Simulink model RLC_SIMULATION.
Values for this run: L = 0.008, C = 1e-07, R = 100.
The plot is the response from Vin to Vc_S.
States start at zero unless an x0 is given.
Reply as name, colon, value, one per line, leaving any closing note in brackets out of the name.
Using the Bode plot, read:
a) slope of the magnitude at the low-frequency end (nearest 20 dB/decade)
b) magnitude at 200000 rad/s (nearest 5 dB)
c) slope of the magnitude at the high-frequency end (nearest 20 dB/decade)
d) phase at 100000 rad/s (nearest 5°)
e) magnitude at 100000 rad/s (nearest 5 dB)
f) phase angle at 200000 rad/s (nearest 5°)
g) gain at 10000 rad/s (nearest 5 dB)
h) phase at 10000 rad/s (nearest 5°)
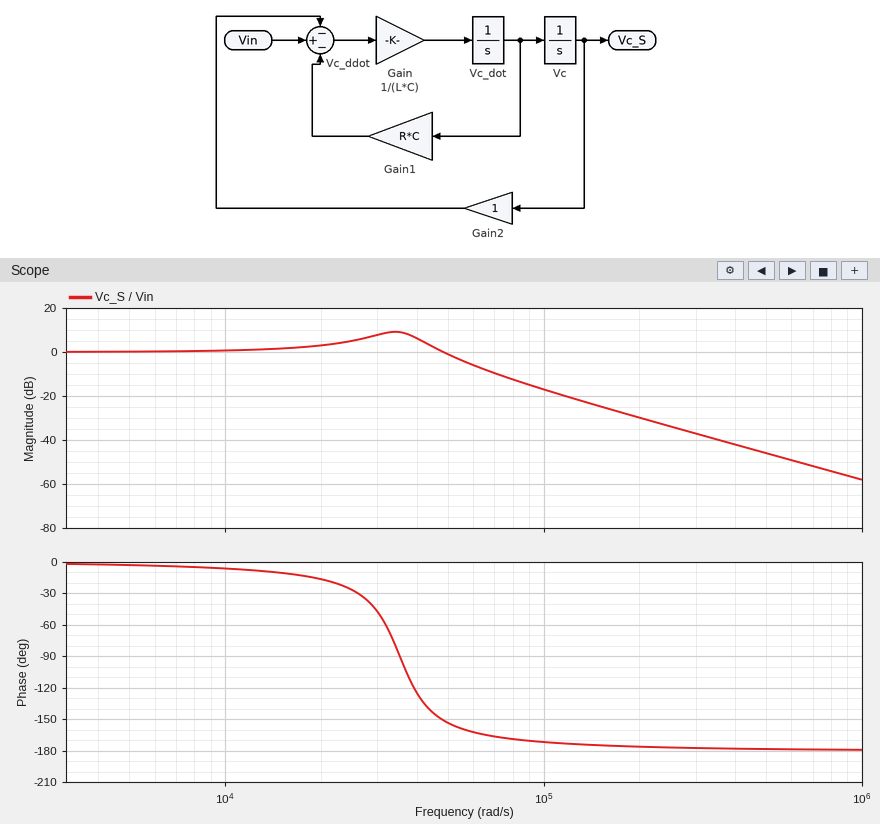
slope of the magnitude at the low-frequency end: 0 dB/decade
magnitude at 200000 rad/s: -30 dB
slope of the magnitude at the high-frequency end: -40 dB/decade
phase at 100000 rad/s: -170°
magnitude at 100000 rad/s: -15 dB
phase angle at 200000 rad/s: -175°
gain at 10000 rad/s: 0 dB
phase at 10000 rad/s: -5°
